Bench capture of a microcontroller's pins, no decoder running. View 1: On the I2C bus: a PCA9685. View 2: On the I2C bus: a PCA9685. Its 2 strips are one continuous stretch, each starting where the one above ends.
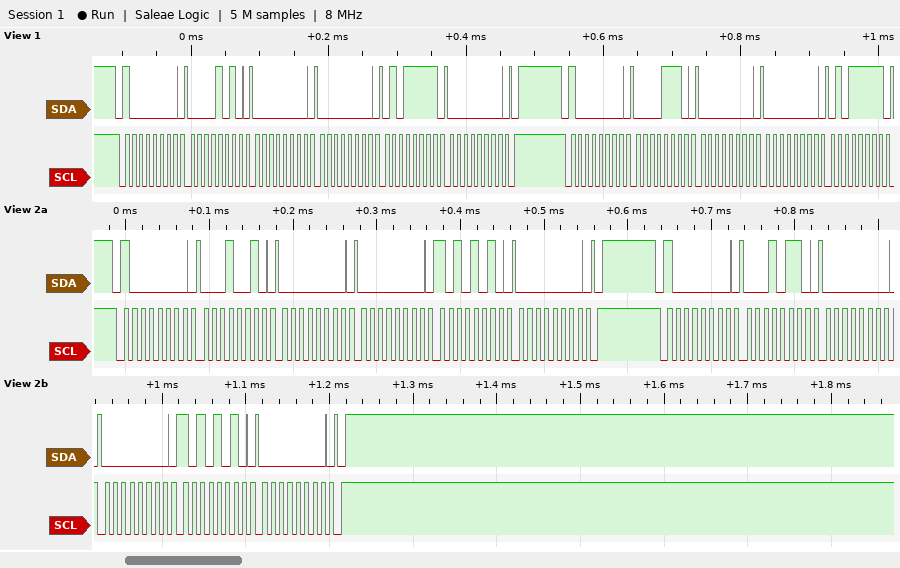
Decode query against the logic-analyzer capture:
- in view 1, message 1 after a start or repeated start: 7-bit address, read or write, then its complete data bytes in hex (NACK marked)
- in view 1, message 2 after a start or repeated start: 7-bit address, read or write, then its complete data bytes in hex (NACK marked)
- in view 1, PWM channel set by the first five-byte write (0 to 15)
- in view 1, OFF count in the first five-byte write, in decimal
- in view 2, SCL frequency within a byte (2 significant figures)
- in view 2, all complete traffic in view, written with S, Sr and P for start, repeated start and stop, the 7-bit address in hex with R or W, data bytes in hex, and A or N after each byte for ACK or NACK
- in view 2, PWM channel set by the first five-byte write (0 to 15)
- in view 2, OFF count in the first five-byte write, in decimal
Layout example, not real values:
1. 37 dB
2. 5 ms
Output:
1. 0x40 write: 0A 00 00 5F 00
2. 0x40 write: 0E 00 00 5F
3. 1
4. 95
5. 100 kHz
6. S 40W A 12 A 00 A 00 A AA A 00 A P S 40W A 16 A 00 A 00 A AA A 00 A P
7. 3
8. 170
